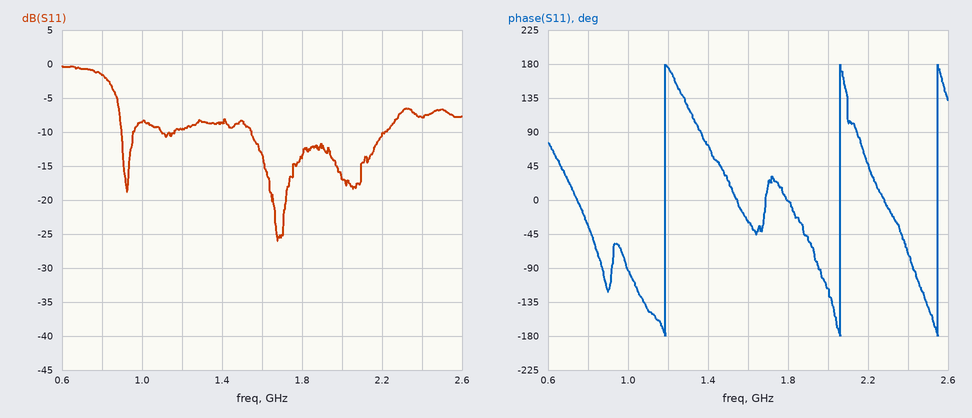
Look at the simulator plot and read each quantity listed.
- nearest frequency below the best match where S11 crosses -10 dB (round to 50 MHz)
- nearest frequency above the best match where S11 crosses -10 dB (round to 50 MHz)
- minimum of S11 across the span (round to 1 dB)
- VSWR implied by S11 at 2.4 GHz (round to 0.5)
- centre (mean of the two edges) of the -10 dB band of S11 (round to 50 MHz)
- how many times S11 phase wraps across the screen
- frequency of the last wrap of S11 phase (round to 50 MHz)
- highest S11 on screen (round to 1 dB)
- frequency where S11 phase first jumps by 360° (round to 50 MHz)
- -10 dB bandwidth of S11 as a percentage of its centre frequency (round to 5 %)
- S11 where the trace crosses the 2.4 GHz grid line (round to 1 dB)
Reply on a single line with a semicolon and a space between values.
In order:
1.55 GHz; 2.20 GHz; -26 dB; 2.5; 1.90 GHz; 3; 2.55 GHz; 0 dB; 1.20 GHz; 35 %; -8 dB
